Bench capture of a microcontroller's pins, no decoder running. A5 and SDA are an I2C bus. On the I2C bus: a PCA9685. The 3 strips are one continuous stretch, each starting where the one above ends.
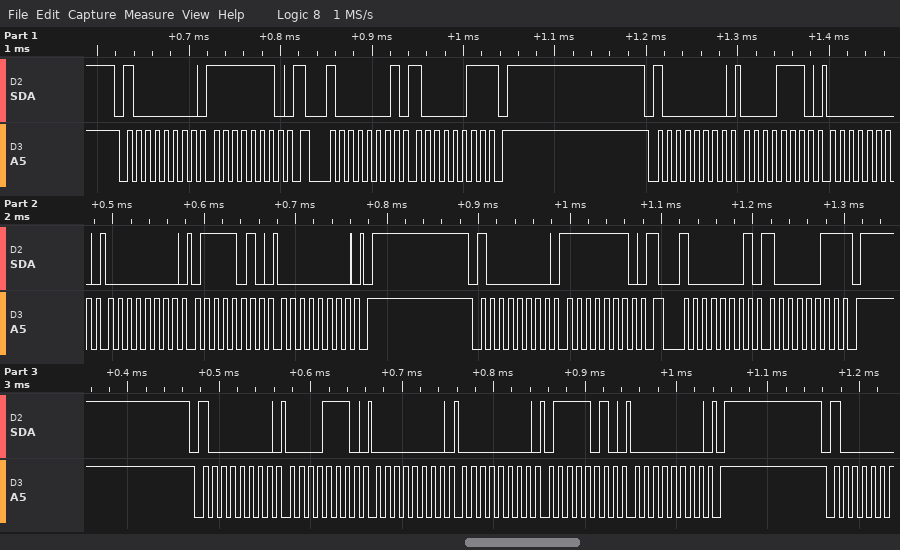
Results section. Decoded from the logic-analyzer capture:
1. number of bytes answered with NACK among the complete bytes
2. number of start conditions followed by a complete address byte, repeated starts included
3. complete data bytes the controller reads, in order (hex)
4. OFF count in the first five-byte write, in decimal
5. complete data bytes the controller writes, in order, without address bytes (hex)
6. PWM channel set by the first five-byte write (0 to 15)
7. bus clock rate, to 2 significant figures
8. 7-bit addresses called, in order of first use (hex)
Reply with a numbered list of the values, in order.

1. 2
2. 6
3. 83 83
4. 122
5. FE 0E 00 00 7A 00 FE 0E 00 00 7A 00
6. 2
7. 100 kHz
8. 0x40
